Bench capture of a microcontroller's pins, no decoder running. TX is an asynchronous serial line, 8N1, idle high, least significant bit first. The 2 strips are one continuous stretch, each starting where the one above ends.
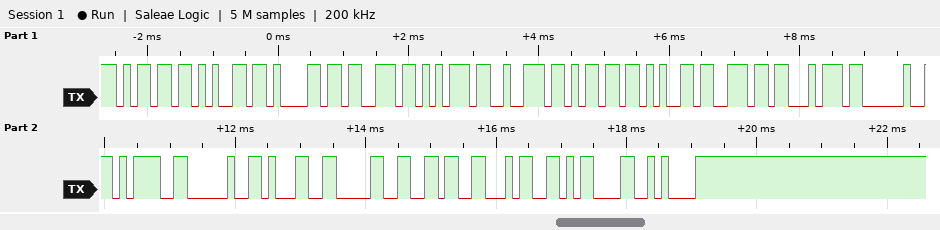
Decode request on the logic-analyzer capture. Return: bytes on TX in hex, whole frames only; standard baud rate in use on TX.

0x6D 0x65 0x61 0x73 0x75 0x72 0x6D 0x65 0x6E 0x74 0x20 0x3D 0x20 0x31 0x30 0x36 0x34 0x0D 0x0A
9600 baud
